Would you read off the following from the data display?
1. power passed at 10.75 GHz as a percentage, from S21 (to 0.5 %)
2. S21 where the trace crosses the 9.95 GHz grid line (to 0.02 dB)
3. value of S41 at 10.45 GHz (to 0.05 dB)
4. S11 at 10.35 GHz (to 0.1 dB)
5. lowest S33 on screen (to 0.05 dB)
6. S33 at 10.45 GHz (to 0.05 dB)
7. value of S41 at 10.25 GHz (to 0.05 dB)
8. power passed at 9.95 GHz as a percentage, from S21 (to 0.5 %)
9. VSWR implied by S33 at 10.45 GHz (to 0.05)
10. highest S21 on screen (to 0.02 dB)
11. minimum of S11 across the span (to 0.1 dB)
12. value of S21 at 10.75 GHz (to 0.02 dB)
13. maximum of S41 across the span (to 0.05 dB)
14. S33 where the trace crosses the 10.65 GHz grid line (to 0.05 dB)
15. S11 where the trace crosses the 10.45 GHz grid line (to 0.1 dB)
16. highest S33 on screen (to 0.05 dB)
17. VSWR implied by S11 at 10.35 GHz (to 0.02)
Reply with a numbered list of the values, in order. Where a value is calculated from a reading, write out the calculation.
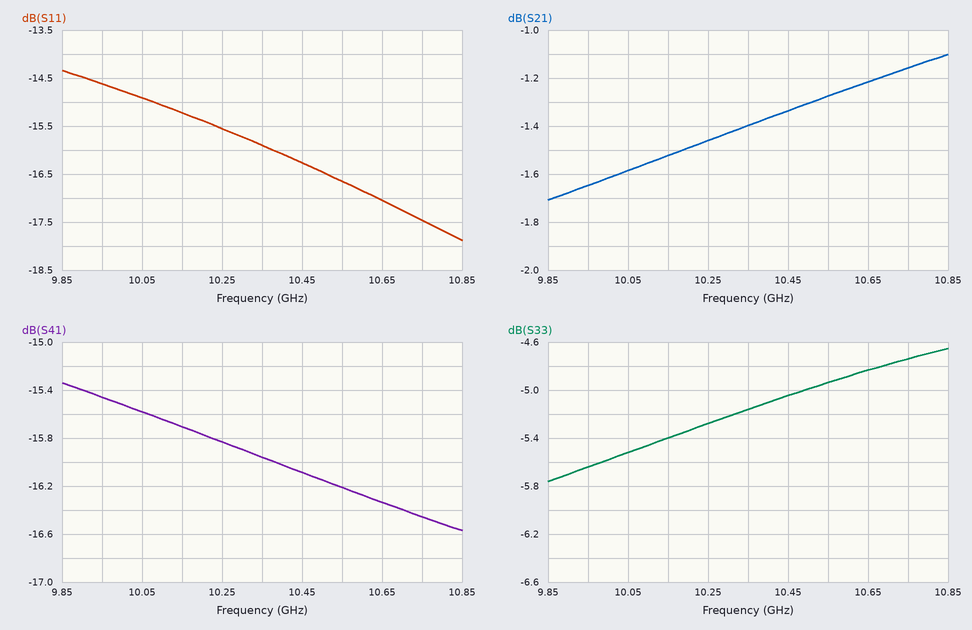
1. 10^(-1.16/10) ≈ 76.6 %, so 76.5 % to the nearest 0.5 %
2. -1.64 dB
3. -16.10 dB
4. -15.9 dB
5. -5.75 dB
6. -5.05 dB
7. -15.85 dB
8. 10^(-1.64/10) ≈ 68.5 %
9. |Γ| = 10^(-5.05/20) = 0.5591; VSWR = (1 + 0.5591)/(1 − 0.5591) ≈ 3.54, so 3.55 to the nearest 0.05
10. -1.10 dB
11. -17.9 dB
12. -1.16 dB
13. -15.35 dB
14. -4.85 dB
15. -16.3 dB
16. -4.65 dB
17. |Γ| = 10^(-15.9/20) = 0.1603; VSWR = (1 + 0.1603)/(1 − 0.1603) ≈ 1.38
